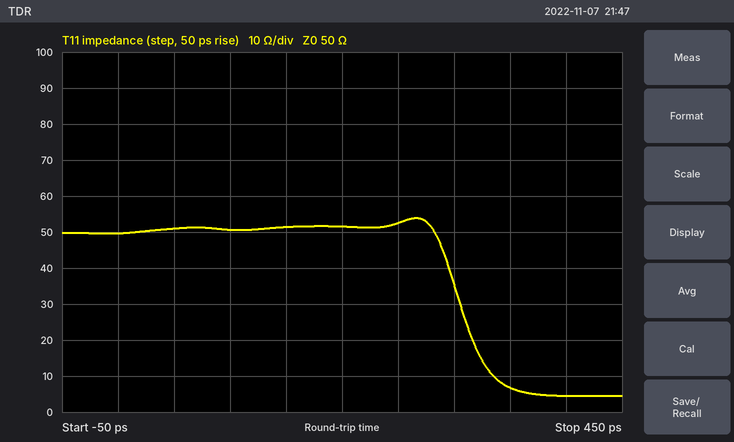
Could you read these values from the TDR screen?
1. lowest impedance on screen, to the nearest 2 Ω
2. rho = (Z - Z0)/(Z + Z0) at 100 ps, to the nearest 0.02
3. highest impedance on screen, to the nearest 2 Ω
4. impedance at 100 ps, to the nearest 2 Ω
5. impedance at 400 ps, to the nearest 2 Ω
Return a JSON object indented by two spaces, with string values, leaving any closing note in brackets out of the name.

{
  "lowest impedance on screen, to the nearest 2 Ω": "4 Ω",
  "rho = (Z - Z0)/(Z + Z0) at 100 ps, to the nearest 0.02": "0.00",
  "highest impedance on screen, to the nearest 2 Ω": "54 Ω",
  "impedance at 100 ps, to the nearest 2 Ω": "50 Ω",
  "impedance at 400 ps, to the nearest 2 Ω": "4 Ω"
}
